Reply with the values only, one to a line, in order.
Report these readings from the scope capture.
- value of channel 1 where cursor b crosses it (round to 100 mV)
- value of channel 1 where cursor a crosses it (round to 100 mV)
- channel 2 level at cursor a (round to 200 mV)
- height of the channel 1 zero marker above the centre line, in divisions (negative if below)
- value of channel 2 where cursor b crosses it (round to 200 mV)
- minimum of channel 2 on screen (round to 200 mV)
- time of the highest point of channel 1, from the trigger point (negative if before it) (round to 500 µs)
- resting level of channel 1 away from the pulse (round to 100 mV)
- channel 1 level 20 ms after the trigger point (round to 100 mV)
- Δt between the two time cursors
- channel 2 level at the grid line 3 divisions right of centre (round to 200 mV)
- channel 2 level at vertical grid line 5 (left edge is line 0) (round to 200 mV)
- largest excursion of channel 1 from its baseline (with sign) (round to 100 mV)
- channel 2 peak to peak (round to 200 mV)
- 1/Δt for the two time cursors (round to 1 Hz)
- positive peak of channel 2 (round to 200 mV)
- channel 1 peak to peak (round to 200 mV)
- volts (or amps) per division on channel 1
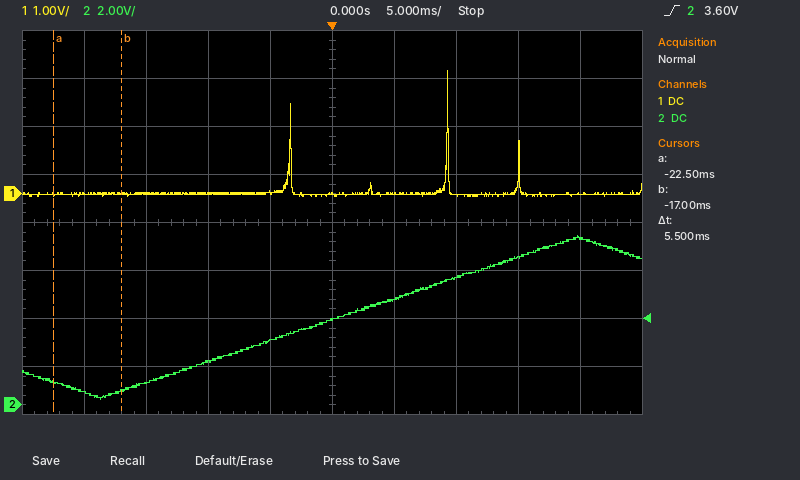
0.0 V
0.0 V
1.0 V
+0.6 div
600 mV
200 mV
+9.5 ms
0.0 V
0.0 V
5.5 ms
6.2 V
3.6 V
+2.6 V
6.8 V
182 Hz
7.0 V
2.6 V
1 V
